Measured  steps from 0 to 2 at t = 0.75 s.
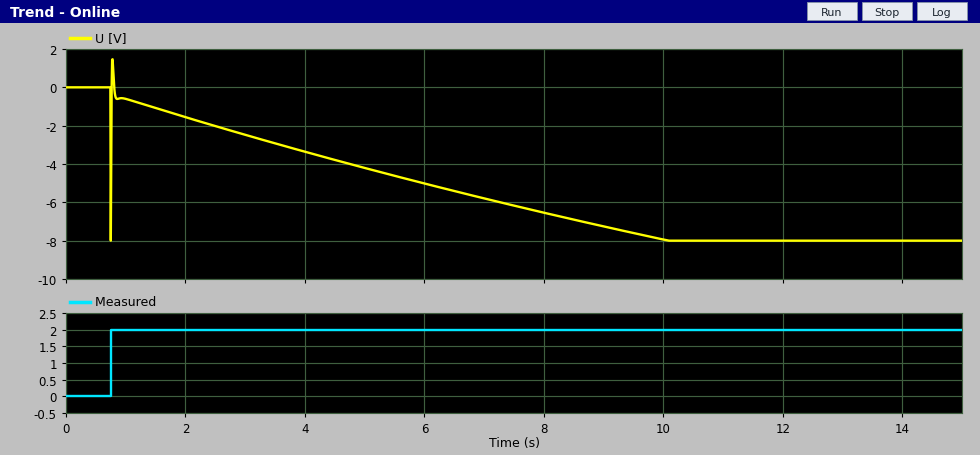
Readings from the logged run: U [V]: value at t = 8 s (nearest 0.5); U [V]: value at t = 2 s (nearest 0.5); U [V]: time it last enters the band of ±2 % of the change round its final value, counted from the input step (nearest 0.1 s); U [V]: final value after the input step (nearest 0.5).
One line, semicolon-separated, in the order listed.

-6.5; -1.5; 9.1 s; -8.0
